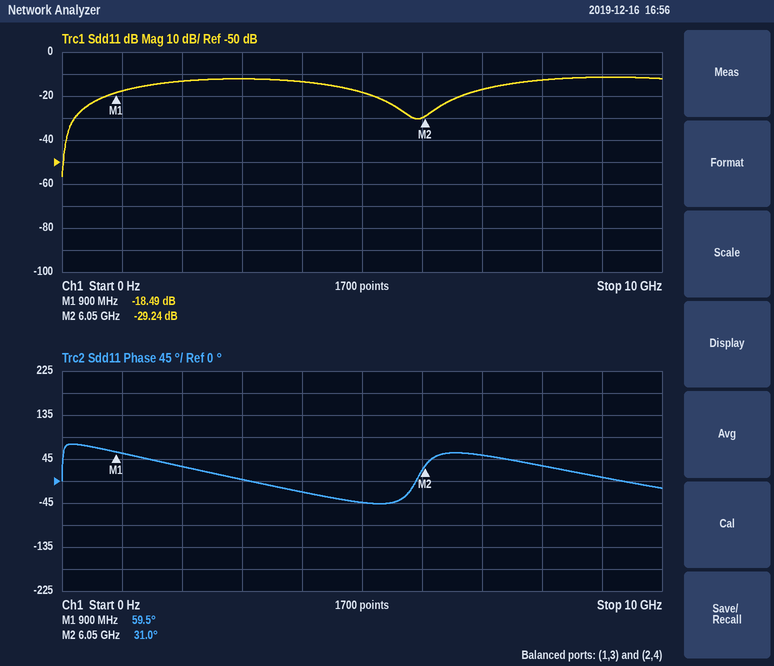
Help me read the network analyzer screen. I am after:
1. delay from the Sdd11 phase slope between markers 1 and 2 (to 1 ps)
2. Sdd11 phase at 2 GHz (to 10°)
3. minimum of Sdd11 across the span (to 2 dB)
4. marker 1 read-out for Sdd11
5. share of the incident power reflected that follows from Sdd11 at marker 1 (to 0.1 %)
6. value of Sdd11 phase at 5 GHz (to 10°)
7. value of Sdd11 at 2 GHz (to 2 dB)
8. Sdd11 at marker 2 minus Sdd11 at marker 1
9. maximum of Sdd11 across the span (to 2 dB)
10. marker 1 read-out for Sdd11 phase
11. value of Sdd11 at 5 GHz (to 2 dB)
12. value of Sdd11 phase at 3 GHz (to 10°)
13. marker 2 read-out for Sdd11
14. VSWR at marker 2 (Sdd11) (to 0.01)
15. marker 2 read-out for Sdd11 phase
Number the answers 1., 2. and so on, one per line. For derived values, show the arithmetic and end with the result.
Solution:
1. −(31° − (59.5°))/(360° × 5.15 GHz) ≈ 15 ps
2. 30°
3. -56 dB
4. -18.49 dB
5. 10^(-18.49/10) ≈ 1.4 %
6. -40°
7. -14 dB
8. -29.24 − (-18.49) = -10.75 dB
9. -12 dB
10. 59.5°
11. -18 dB
12. 0°
13. -29.24 dB
14. (1 + 0.0345)/(1 − 0.0345) ≈ 1.07
15. 31.0°
